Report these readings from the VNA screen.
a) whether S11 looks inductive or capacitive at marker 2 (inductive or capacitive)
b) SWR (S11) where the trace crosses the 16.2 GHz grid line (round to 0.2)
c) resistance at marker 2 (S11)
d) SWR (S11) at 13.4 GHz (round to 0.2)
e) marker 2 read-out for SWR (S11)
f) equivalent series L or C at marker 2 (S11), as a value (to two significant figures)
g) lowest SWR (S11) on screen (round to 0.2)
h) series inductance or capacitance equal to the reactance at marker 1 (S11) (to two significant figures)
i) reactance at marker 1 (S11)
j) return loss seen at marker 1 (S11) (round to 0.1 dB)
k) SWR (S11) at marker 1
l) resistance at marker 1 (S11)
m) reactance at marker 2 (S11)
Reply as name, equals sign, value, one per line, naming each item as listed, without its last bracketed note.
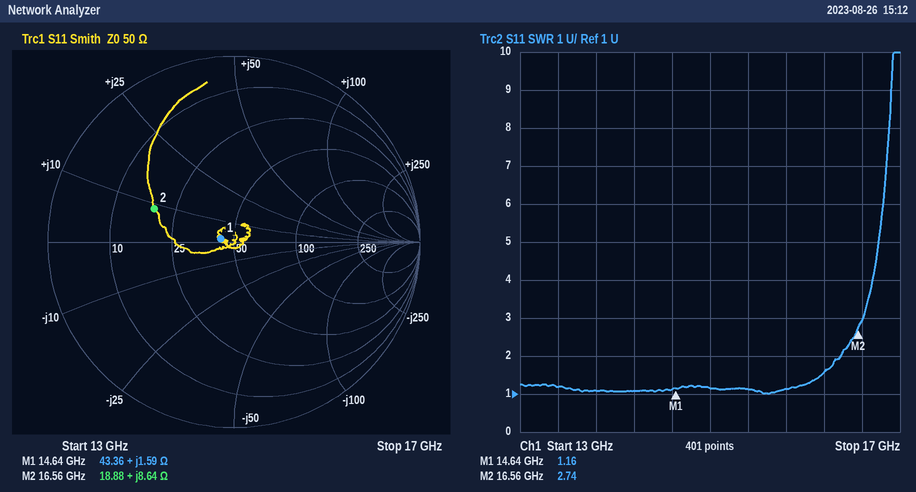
whether S11 looks inductive or capacitive at marker 2 = inductive
SWR (S11) where the trace crosses the 16.2 GHz grid line = 1.6
resistance at marker 2 = 18.88 Ω
SWR (S11) at 13.4 GHz = 1.2
marker 2 read-out for SWR = 2.74
equivalent series L or C at marker 2 (S11), as a value = 83 pH
lowest SWR (S11) on screen = 1.0
series inductance or capacitance equal to the reactance at marker 1 (S11) = 17 pH
reactance at marker 1 = +1.59 Ω
return loss seen at marker 1 (S11) = 22.7 dB
SWR (S11) at marker 1 = 1.16
resistance at marker 1 = 43.36 Ω
reactance at marker 2 = +8.64 Ω
